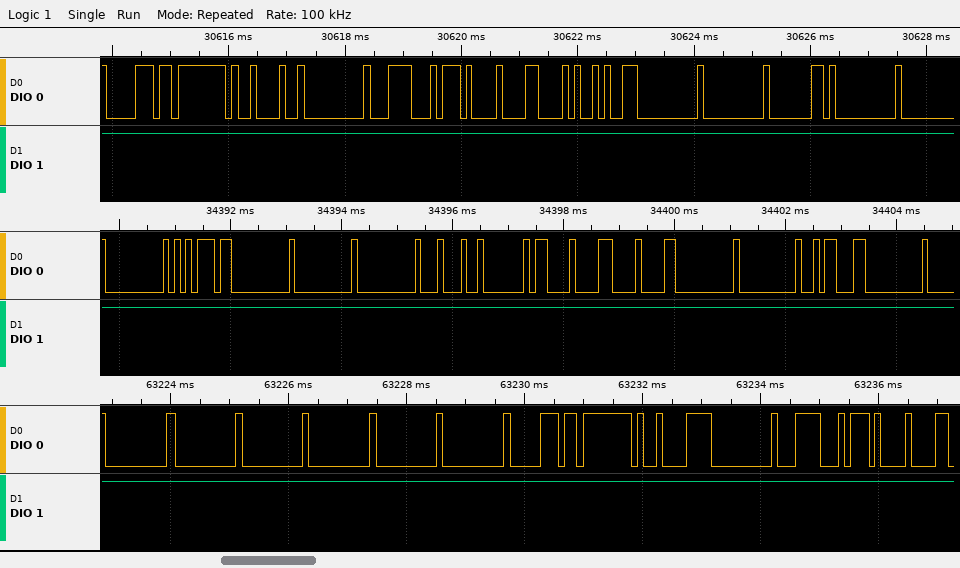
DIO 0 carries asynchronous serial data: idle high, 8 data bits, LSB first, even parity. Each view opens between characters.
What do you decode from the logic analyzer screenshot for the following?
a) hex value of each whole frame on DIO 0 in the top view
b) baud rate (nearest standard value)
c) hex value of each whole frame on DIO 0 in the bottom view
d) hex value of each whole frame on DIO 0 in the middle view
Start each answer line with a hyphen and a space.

- 70, FF, 42, 00, 3C, 17, 18, 29, 00, 00, C0, 00
- 9600 baud
- 00, 00, 00, 00, 00, 00, 70, FF, C2, 00, 3C, 17
- 00, 75, 00, 00, 00, 44, 40, 08, 08, 00, 00, 1A, 00
